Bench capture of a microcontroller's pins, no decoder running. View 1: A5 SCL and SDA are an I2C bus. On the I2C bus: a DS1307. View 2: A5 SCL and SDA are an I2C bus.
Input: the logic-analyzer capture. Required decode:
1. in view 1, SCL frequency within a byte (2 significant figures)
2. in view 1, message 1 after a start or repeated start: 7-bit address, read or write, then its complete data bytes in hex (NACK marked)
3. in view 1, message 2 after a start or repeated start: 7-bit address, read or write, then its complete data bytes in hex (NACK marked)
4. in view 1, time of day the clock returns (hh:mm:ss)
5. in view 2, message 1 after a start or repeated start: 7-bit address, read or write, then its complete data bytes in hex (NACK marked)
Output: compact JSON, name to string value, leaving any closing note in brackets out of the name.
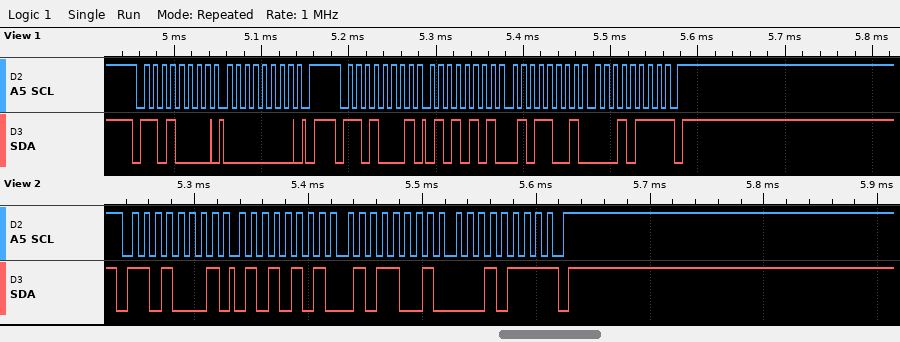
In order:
{"in view 1, SCL frequency within a byte": "100 kHz", "in view 1, message 1 after a start or repeated start: 7-bit address, read or write, then its complete data bytes in hex": "0x68 write: 00", "in view 1, message 2 after a start or repeated start: 7-bit address, read or write, then its complete data bytes in hex": "0x68 read: 55 59 17 NACK", "in view 1, time of day the clock returns": "17:59:55", "in view 2, message 1 after a start or repeated start: 7-bit address, read or write, then its complete data bytes in hex": "0x68 read: 55 59 17 NACK"}
